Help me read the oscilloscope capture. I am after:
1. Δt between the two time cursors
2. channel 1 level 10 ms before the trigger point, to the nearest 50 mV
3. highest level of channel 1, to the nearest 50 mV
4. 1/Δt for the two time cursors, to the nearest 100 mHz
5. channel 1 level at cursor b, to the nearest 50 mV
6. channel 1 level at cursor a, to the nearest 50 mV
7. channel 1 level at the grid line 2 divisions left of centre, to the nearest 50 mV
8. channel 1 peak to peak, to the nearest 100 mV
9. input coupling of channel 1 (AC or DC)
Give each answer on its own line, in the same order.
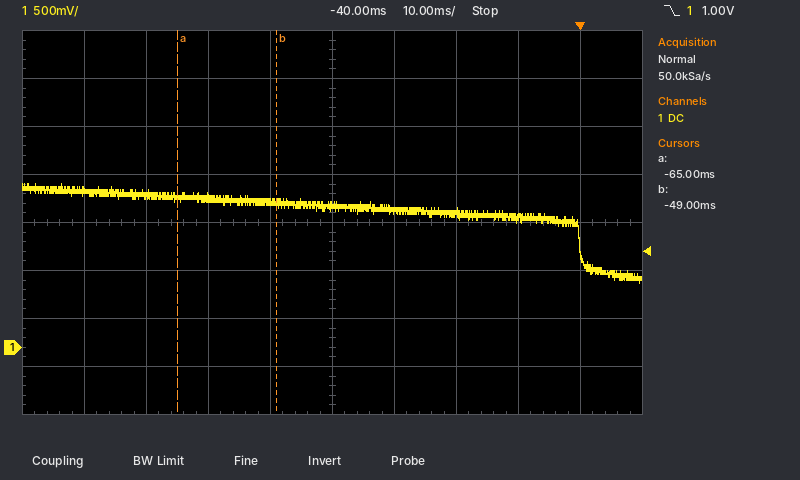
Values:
16 ms
1.35 V
1.70 V
62.5 Hz
1.50 V
1.55 V
1.55 V
1.00 V
DC
